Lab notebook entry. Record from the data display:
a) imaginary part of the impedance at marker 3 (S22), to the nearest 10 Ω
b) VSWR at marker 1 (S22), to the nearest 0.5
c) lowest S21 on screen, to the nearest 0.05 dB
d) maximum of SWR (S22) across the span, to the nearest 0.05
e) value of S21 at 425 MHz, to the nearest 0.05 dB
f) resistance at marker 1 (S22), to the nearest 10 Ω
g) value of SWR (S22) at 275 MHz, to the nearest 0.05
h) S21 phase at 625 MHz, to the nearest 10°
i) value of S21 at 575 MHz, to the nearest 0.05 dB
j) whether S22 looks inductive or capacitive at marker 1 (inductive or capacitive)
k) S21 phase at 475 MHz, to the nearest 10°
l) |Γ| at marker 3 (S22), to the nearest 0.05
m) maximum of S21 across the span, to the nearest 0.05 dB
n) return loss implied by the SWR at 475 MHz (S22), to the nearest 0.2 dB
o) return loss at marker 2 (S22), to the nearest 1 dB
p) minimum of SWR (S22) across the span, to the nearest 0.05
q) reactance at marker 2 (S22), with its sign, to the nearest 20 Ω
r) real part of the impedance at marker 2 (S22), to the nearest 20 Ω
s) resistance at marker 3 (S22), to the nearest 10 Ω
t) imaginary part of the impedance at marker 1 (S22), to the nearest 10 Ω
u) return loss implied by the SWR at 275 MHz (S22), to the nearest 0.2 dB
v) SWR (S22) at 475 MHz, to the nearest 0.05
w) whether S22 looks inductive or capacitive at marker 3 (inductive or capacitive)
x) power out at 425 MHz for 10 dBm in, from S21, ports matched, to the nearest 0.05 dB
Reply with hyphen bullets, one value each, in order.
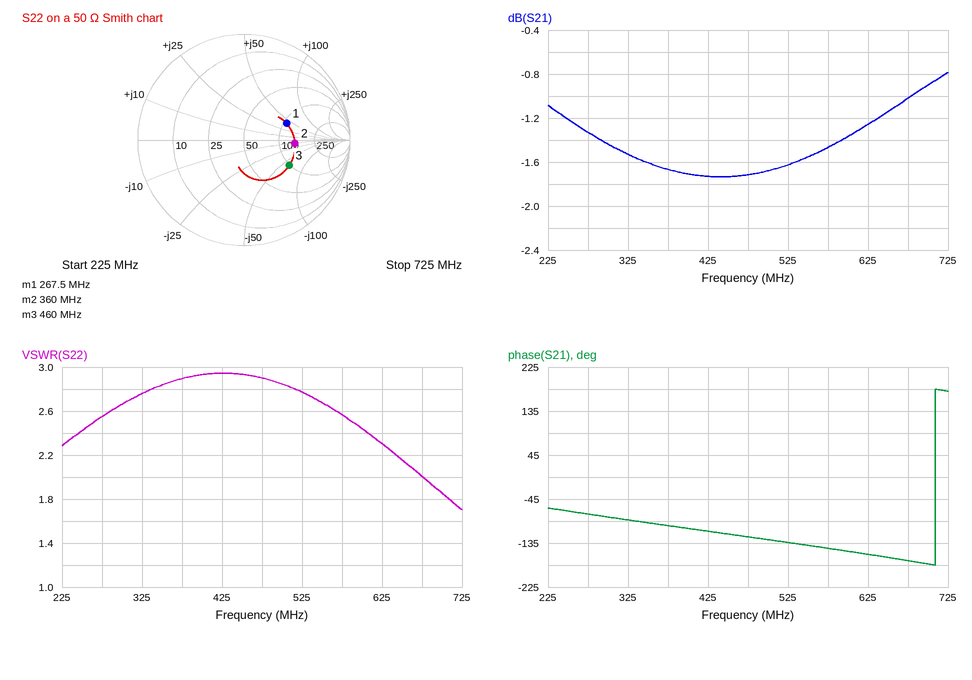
- -60 Ω
- 2.5
- -1.75 dB
- 2.95
- -1.75 dB
- 110 Ω
- 2.55
- -160°
- -1.45 dB
- inductive
- -120°
- 0.50
- -0.80 dB
- 6.2 dB
- 6 dB
- 1.70
- -20 Ω
- 140 Ω
- 100 Ω
- +40 Ω
- 7.2 dB
- 2.90
- capacitive
- 8.25 dBm
